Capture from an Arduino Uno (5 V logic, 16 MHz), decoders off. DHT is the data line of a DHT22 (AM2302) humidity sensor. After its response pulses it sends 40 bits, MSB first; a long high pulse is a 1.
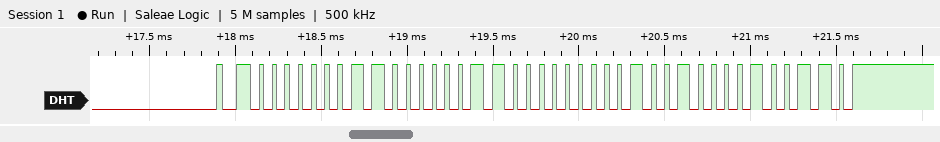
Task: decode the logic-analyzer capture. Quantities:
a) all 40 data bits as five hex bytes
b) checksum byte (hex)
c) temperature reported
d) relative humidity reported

01 81 80 24 26
0x26
-3.6 °C
38.5 %
